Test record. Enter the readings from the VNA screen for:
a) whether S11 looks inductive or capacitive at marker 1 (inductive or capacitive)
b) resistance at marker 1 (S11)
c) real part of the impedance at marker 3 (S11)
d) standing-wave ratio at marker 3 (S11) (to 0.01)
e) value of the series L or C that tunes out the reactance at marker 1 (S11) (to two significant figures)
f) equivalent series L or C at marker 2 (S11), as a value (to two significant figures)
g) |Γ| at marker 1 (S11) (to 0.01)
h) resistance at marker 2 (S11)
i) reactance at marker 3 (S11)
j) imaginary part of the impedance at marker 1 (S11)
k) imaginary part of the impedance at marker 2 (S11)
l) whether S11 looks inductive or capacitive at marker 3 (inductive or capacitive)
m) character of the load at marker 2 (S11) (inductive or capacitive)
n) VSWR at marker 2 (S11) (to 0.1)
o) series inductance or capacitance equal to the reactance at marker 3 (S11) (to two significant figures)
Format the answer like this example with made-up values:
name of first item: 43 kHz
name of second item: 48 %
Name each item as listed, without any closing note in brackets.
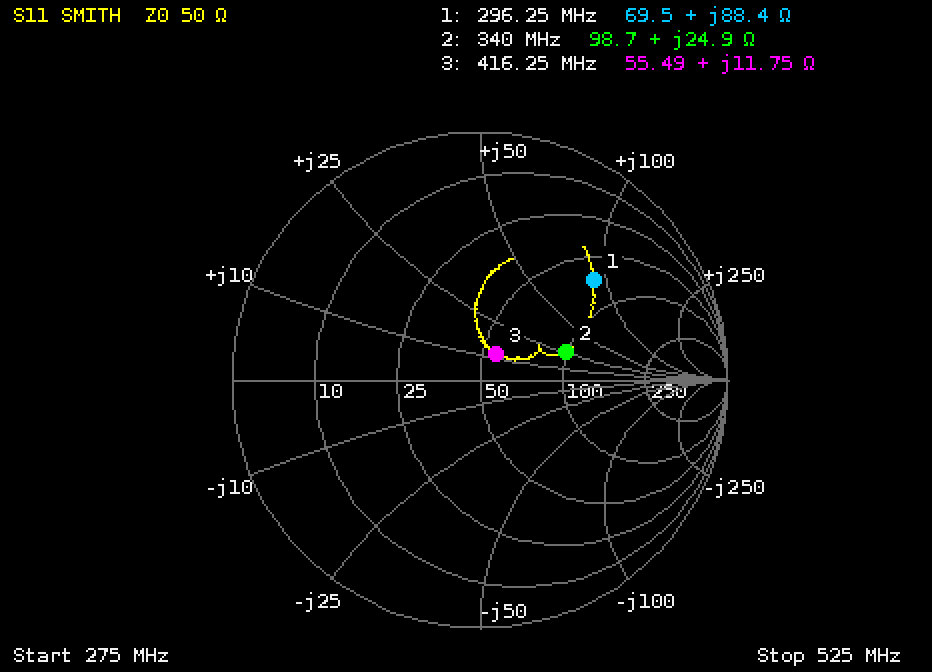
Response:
whether S11 looks inductive or capacitive at marker 1: inductive
resistance at marker 1: 69.5 Ω
real part of the impedance at marker 3: 55.49 Ω
standing-wave ratio at marker 3 (S11): 1.28
value of the series L or C that tunes out the reactance at marker 1 (S11): 6.1 pF
equivalent series L or C at marker 2 (S11), as a value: 12 nH
|Γ| at marker 1 (S11): 0.61
resistance at marker 2: 98.7 Ω
reactance at marker 3: +11.75 Ω
imaginary part of the impedance at marker 1: +88.4 Ω
imaginary part of the impedance at marker 2: +24.9 Ω
whether S11 looks inductive or capacitive at marker 3: inductive
character of the load at marker 2 (S11): inductive
VSWR at marker 2 (S11): 2.1
series inductance or capacitance equal to the reactance at marker 3 (S11): 4.5 nH
